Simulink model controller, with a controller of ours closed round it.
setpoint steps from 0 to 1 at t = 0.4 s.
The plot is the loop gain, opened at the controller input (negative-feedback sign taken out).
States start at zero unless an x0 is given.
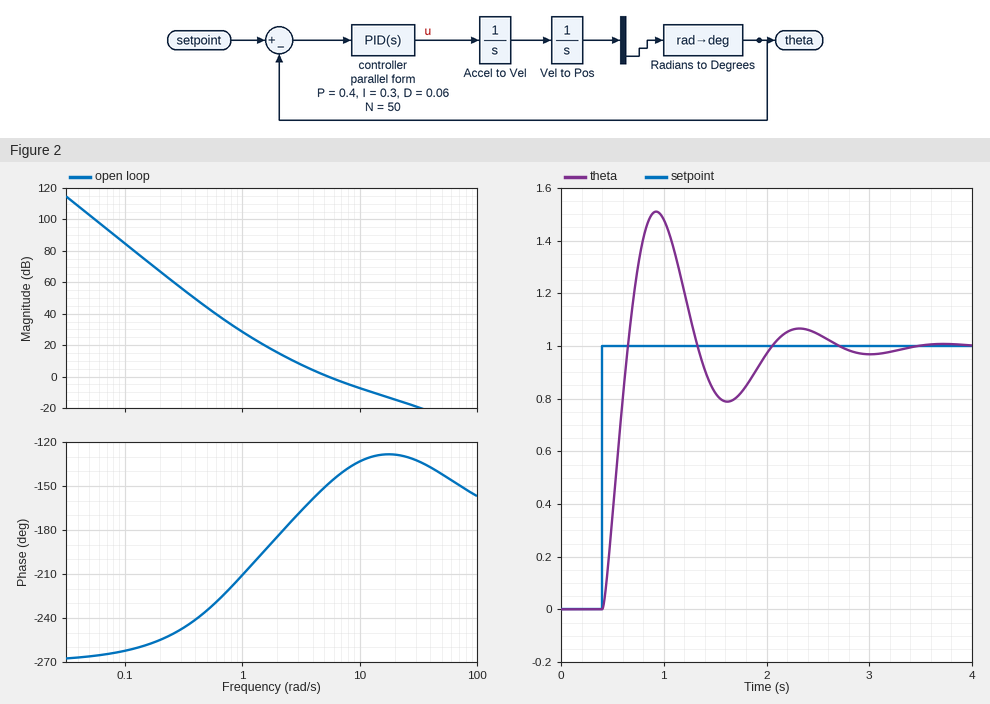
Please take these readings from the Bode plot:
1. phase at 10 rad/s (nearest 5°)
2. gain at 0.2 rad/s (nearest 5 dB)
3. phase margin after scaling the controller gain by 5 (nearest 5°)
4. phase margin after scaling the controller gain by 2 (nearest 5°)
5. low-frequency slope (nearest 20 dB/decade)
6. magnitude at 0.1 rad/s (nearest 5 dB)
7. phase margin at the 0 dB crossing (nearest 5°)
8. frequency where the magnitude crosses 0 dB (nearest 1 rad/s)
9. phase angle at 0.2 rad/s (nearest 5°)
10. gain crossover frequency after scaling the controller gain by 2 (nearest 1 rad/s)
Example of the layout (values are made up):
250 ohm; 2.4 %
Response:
-135°; 65 dB; 50°; 45°; -60 dB/decade; 85 dB; 30°; 5 rad/s; -255°; 9 rad/s
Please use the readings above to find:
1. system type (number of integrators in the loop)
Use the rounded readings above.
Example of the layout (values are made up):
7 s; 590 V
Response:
3
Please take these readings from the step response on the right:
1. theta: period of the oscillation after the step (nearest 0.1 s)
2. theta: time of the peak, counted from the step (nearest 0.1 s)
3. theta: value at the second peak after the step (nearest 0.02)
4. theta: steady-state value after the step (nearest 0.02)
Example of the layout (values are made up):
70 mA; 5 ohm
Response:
1.4 s; 0.5 s; 1.06; 1.00
